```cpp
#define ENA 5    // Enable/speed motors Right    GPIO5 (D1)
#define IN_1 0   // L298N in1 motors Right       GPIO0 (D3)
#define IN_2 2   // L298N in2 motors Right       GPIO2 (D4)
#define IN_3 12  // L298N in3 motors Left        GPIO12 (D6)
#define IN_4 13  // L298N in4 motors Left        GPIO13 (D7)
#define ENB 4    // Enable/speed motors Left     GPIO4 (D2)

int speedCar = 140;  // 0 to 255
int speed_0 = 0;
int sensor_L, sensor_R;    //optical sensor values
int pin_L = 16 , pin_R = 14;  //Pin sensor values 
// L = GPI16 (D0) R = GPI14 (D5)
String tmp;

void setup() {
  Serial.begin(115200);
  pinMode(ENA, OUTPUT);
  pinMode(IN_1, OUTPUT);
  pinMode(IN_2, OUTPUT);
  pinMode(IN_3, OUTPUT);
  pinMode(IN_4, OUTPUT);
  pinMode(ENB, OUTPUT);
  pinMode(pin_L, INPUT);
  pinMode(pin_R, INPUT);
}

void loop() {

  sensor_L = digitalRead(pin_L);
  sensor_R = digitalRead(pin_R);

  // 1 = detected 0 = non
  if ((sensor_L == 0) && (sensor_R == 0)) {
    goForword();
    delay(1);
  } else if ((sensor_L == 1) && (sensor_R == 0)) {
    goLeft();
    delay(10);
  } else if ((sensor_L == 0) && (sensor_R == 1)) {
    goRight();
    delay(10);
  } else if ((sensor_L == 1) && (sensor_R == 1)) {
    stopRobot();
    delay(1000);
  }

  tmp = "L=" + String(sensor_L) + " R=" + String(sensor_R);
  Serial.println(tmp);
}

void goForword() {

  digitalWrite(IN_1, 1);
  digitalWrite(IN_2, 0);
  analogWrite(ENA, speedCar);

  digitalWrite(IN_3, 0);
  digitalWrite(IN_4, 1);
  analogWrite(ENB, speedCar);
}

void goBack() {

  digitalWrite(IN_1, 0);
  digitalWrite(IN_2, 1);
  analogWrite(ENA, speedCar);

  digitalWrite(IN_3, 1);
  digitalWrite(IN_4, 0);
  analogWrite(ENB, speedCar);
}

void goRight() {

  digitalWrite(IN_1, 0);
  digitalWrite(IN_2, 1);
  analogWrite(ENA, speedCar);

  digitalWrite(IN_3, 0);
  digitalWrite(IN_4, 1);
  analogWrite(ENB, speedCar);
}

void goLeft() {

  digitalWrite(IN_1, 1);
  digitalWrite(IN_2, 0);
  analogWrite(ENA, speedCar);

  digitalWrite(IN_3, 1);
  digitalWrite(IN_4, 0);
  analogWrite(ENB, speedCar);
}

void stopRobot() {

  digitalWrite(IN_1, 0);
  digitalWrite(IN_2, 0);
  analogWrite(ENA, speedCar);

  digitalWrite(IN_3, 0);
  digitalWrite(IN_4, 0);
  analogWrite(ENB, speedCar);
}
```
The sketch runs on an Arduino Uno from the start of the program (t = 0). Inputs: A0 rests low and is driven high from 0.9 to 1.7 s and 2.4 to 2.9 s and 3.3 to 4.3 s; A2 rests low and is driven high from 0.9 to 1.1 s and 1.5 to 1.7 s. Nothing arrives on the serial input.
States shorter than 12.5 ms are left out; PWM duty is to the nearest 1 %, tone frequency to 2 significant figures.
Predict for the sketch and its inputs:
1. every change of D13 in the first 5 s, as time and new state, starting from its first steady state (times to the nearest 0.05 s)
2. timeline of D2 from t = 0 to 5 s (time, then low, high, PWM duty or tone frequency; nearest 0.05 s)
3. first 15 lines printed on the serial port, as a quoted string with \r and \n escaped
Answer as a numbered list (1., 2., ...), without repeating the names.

1. 0 s high; 0.9 s low; 1.9 s high
2. 0 s low; 2.4 s high; 2.9 s low; 3.3 s high; 4.3 s low
3. "L=0 R=0\r\nL=0 R=0\r\nL=0 R=0\r\nL=0 R=0\r\nL=0 R=0\r\nL=0 R=0\r\nL=0 R=0\r\nL=0 R=0\r\nL=0 R=0\r\nL=0 R=0\r\nL=0 R=0\r\nL=0 R=0\r\nL=0 R=0\r\nL=0 R=0\r\nL=0 R=0\r\n"
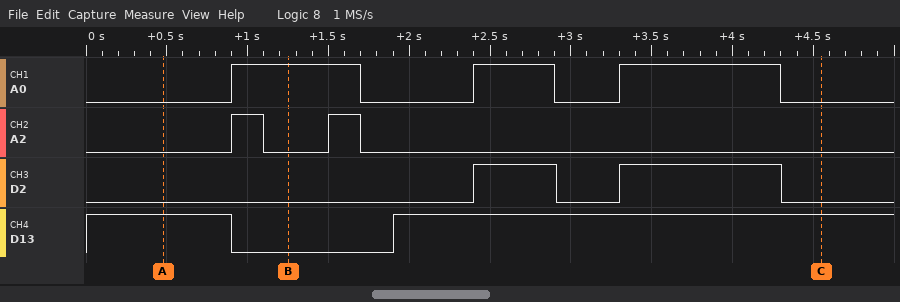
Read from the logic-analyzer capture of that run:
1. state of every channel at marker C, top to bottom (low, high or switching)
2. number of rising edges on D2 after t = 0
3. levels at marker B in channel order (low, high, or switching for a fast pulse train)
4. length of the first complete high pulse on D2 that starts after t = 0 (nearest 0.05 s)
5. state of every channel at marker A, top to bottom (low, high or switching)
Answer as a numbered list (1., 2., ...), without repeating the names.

1. A0 low, A2 low, D2 low, D13 high
2. 2
3. A0 high, A2 low, D2 low, D13 low
4. 0.50 s
5. A0 low, A2 low, D2 low, D13 high
